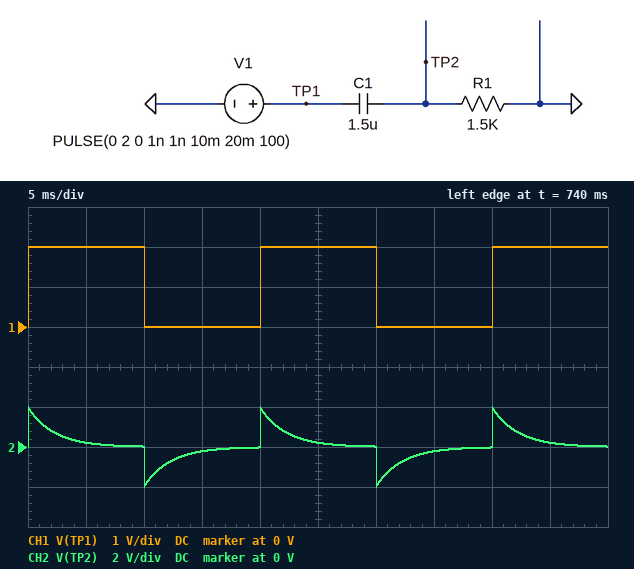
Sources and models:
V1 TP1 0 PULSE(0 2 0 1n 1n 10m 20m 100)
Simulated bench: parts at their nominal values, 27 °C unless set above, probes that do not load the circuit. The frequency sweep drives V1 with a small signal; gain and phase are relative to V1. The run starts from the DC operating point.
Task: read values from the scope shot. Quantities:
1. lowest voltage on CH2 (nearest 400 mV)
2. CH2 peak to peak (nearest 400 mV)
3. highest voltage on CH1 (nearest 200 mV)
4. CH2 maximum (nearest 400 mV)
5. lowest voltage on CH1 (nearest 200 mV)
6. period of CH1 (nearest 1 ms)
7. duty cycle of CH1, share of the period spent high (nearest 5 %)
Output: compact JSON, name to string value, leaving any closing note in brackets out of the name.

{"lowest voltage on CH2": "-2.0 V", "CH2 peak to peak": "4.0 V", "highest voltage on CH1": "2.0 V", "CH2 maximum": "2.0 V", "lowest voltage on CH1": "0 V", "period of CH1": "20 ms", "duty cycle of CH1, share of the period spent high": "50 %"}
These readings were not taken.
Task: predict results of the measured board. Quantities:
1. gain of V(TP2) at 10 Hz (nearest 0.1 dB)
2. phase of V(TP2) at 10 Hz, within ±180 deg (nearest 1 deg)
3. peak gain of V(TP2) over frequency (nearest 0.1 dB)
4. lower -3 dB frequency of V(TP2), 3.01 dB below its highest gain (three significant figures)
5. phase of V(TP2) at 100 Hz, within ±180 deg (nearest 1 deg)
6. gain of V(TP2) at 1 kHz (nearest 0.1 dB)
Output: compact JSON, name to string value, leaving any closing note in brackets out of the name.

{"gain of V(TP2) at 10 Hz": "-17.1 dB", "phase of V(TP2) at 10 Hz, within ±180 deg": "82 deg", "peak gain of V(TP2) over frequency": "0 dB", "lower -3 dB frequency of V(TP2), 3.01 dB below its highest gain": "70.7 Hz", "phase of V(TP2) at 100 Hz, within ±180 deg": "35 deg", "gain of V(TP2) at 1 kHz": "0 dB"}
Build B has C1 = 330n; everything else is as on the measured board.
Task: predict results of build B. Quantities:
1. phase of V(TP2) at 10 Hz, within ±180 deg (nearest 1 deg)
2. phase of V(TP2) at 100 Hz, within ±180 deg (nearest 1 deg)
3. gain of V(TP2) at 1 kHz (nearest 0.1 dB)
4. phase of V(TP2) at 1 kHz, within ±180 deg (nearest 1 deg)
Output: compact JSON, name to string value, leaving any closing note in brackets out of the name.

{"phase of V(TP2) at 10 Hz, within ±180 deg": "88 deg", "phase of V(TP2) at 100 Hz, within ±180 deg": "73 deg", "gain of V(TP2) at 1 kHz": "-0.4 dB", "phase of V(TP2) at 1 kHz, within ±180 deg": "18 deg"}
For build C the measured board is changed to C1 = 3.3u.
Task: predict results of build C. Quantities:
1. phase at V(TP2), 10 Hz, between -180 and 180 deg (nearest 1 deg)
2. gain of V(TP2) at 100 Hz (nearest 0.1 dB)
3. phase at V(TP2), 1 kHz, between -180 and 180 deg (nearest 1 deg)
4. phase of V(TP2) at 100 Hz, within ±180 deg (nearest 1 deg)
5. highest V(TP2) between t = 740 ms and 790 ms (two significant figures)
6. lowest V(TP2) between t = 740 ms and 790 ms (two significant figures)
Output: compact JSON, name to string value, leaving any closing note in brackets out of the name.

{"phase at V(TP2), 10 Hz, between -180 and 180 deg": "73 deg", "gain of V(TP2) at 100 Hz": "-0.4 dB", "phase at V(TP2), 1 kHz, between -180 and 180 deg": "2 deg", "phase of V(TP2) at 100 Hz, within ±180 deg": "18 deg", "highest V(TP2) between t = 740 ms and 790 ms": "1.8 V", "lowest V(TP2) between t = 740 ms and 790 ms": "-1.8 V"}
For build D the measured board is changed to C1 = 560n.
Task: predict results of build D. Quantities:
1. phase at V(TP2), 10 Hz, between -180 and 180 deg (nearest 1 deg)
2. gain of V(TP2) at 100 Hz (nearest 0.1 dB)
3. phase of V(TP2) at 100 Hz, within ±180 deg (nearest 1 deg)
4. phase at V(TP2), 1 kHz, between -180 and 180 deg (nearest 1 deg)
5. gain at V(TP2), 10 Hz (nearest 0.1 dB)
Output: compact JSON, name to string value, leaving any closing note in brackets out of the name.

{"phase at V(TP2), 10 Hz, between -180 and 180 deg": "87 deg", "gain of V(TP2) at 100 Hz": "-6.6 dB", "phase of V(TP2) at 100 Hz, within ±180 deg": "62 deg", "phase at V(TP2), 1 kHz, between -180 and 180 deg": "11 deg", "gain at V(TP2), 10 Hz": "-25.6 dB"}
